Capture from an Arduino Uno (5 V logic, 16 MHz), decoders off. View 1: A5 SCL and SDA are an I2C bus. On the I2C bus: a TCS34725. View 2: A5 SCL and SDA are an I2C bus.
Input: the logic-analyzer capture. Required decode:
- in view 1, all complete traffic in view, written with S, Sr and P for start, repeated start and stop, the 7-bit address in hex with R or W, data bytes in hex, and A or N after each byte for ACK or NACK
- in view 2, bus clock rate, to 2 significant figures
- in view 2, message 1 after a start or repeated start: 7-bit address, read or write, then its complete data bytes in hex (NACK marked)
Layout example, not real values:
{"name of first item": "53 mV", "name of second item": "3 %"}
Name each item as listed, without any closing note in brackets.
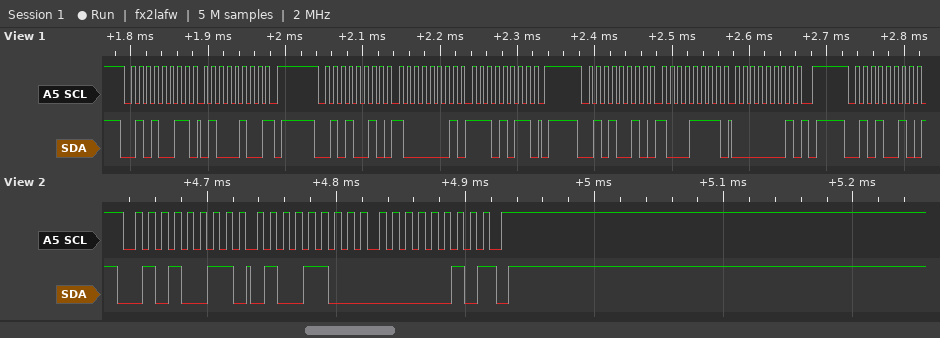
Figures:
{"in view 1, all complete traffic in view, written with S, Sr and P for start, repeated start and stop, the 7-bit address in hex with R or W, data bytes in hex, and A or N after each byte for ACK or NACK": "S 29R A 44 N P S 29W A 81 A EB A P S 29W A 8F A 01 A P S 29W A", "in view 2, bus clock rate, to 2 significant figures": "100 kHz", "in view 2, message 1 after a start or repeated start: 7-bit address, read or write, then its complete data bytes in hex": "0x29 read: 4C 02 NACK"}
